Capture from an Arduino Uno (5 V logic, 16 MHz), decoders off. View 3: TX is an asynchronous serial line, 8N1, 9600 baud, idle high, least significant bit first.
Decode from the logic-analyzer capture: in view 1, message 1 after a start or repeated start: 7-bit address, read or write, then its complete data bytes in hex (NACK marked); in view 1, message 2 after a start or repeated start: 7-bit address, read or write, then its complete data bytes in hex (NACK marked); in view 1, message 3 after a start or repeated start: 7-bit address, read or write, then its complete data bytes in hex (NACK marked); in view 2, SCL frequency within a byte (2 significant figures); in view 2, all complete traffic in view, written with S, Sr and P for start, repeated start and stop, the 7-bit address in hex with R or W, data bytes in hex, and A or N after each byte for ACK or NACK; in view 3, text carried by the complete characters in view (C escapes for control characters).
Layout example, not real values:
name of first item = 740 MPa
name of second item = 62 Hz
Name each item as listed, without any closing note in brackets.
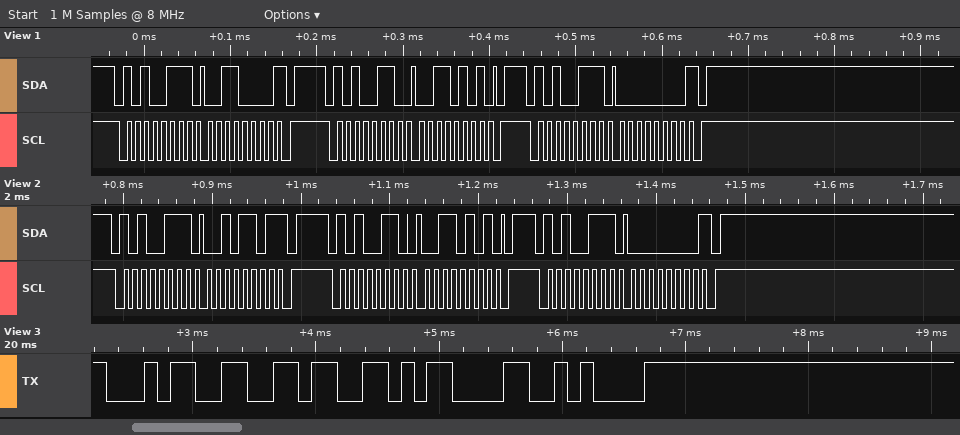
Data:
in view 1, message 1 after a start or repeated start: 7-bit address, read or write, then its complete data bytes in hex = 0x53 read: 30 NACK
in view 1, message 2 after a start or repeated start: 7-bit address, read or write, then its complete data bytes in hex = 0x53 write: 35
in view 1, message 3 after a start or repeated start: 7-bit address, read or write, then its complete data bytes in hex = 0x53 read: 00 NACK
in view 2, SCL frequency within a byte = 100 kHz
in view 2, all complete traffic in view, written with S, Sr and P for start, repeated start and stop, the 7-bit address in hex with R or W, data bytes in hex, and A or N after each byte for ACK or NACK = S 53R A 2D N P S 53W A 35 A P S 53R A 00 N P
in view 3, text carried by the complete characters in view = "46\r\n"
